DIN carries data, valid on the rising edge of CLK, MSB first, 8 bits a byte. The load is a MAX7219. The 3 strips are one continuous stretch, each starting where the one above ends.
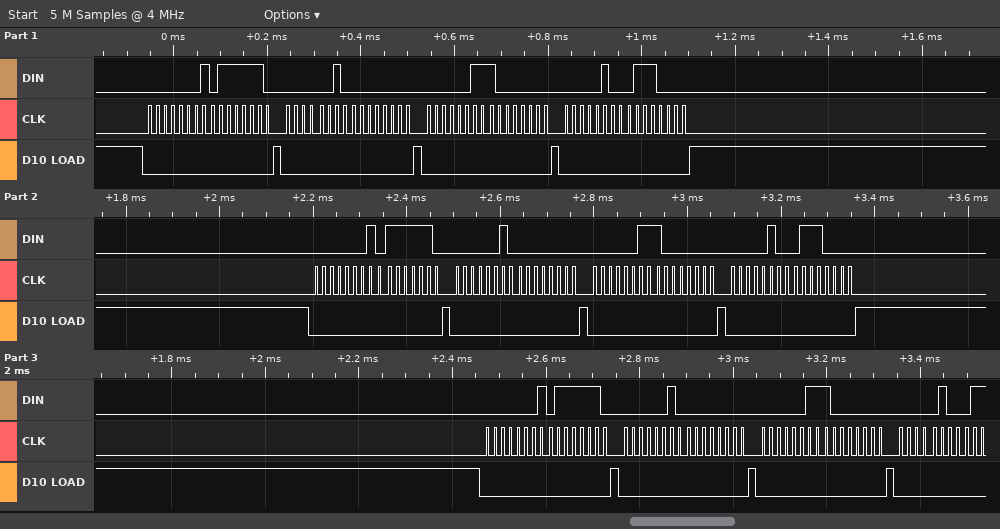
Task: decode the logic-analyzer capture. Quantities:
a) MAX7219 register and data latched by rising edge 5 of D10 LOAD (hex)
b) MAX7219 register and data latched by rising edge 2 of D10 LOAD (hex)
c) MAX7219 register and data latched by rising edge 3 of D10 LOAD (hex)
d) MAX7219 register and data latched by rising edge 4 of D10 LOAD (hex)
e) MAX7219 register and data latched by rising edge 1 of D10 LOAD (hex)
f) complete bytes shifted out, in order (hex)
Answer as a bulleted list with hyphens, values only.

- register 0x1, data 0x7E
- register 0x2, data 0x00
- register 0x3, data 0x80
- register 0x4, data 0x70
- register 0x1, data 0x7E
- 01 7E 02 00 03 80 04 70 01 7E 02 00 03 80 04 70 01 7E 02 00 03 80 04
